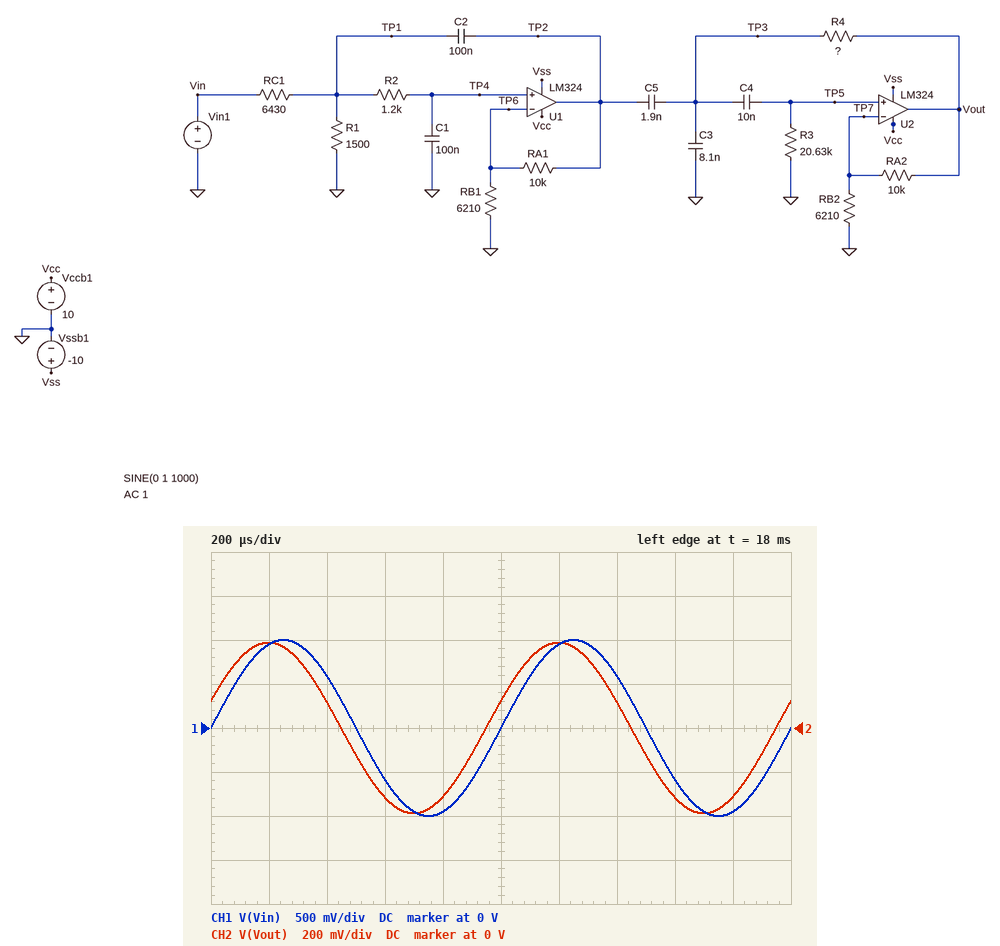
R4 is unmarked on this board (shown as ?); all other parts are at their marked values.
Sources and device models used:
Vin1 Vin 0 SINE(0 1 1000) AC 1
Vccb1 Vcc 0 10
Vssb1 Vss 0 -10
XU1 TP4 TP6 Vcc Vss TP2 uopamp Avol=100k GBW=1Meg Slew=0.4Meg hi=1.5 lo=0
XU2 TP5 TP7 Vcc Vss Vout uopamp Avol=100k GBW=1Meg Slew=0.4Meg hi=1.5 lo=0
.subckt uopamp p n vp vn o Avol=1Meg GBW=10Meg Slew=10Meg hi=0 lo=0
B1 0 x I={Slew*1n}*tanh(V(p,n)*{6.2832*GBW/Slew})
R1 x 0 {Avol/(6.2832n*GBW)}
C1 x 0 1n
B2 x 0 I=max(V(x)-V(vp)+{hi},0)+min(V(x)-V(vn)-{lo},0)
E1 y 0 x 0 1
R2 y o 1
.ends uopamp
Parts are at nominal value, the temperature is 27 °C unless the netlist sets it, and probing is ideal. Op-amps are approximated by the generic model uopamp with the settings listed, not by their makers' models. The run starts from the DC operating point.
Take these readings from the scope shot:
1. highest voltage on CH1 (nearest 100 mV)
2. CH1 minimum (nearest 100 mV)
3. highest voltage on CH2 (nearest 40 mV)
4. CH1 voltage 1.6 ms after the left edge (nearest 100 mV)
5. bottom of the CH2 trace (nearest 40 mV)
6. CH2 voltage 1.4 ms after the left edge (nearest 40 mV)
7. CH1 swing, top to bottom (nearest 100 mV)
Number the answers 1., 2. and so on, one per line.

1. 1.0 V
2. -1.0 V
3. 400 mV
4. -600 mV
5. -400 mV
6. 120 mV
7. 2.0 V
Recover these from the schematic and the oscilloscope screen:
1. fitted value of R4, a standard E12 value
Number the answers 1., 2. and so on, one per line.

1. 47 kΩ
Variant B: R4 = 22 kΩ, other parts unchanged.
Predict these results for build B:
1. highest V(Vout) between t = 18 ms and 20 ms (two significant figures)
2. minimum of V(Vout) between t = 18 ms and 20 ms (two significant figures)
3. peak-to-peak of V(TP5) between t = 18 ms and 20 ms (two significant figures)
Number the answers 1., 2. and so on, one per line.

1. 820 mV
2. -820 mV
3. 630 mV
